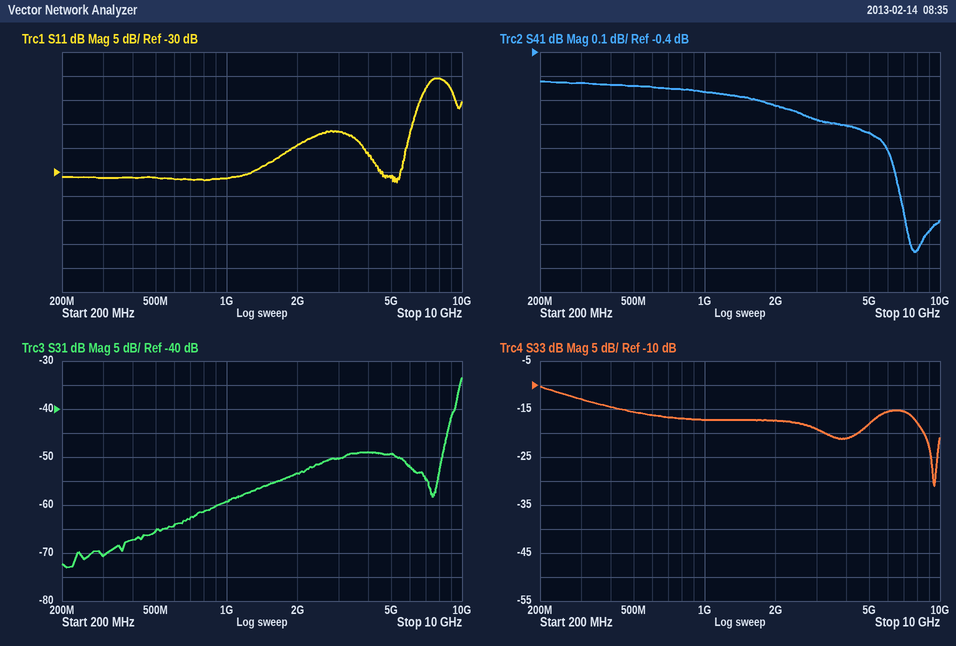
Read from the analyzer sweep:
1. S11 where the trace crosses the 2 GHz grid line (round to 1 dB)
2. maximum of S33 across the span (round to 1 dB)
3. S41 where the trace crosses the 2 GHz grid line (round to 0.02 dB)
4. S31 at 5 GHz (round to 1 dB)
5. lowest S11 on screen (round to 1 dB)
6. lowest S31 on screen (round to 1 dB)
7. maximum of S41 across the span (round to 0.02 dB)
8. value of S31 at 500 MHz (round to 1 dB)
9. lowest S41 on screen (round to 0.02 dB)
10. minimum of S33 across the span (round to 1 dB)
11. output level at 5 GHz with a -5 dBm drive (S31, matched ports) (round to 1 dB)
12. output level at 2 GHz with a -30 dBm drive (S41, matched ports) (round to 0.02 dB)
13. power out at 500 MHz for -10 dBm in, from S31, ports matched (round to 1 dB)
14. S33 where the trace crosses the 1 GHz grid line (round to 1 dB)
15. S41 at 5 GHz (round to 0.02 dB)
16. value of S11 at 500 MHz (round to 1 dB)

-24 dB
-10 dB
-0.62 dB
-49 dB
-32 dB
-73 dB
-0.52 dB
-65 dB
-1.24 dB
-31 dB
-54 dBm
-30.62 dBm
-75 dBm
-17 dB
-0.74 dB
-31 dB
